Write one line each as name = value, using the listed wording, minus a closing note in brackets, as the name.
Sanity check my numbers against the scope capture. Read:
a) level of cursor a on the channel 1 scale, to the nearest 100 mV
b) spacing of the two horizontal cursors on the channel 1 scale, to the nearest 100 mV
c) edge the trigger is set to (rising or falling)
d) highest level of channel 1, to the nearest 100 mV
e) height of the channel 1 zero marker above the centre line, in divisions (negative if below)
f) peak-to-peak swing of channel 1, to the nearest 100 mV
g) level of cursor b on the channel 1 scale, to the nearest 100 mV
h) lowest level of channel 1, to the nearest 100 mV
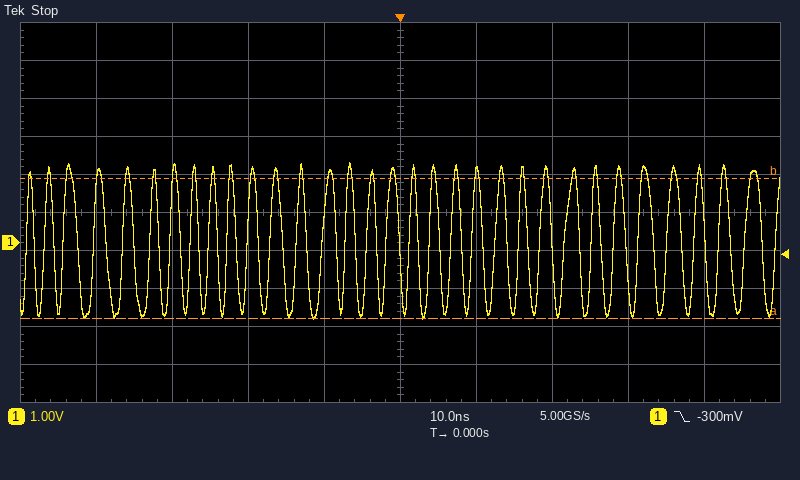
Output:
level of cursor a on the channel 1 scale, to the nearest 100 mV = -2.0 V
spacing of the two horizontal cursors on the channel 1 scale, to the nearest 100 mV = 3.7 V
edge the trigger is set to = falling
highest level of channel 1, to the nearest 100 mV = 2.1 V
height of the channel 1 zero marker above the centre line, in divisions = -0.8 div
peak-to-peak swing of channel 1, to the nearest 100 mV = 4.1 V
level of cursor b on the channel 1 scale, to the nearest 100 mV = 1.7 V
lowest level of channel 1, to the nearest 100 mV = -2.0 V
